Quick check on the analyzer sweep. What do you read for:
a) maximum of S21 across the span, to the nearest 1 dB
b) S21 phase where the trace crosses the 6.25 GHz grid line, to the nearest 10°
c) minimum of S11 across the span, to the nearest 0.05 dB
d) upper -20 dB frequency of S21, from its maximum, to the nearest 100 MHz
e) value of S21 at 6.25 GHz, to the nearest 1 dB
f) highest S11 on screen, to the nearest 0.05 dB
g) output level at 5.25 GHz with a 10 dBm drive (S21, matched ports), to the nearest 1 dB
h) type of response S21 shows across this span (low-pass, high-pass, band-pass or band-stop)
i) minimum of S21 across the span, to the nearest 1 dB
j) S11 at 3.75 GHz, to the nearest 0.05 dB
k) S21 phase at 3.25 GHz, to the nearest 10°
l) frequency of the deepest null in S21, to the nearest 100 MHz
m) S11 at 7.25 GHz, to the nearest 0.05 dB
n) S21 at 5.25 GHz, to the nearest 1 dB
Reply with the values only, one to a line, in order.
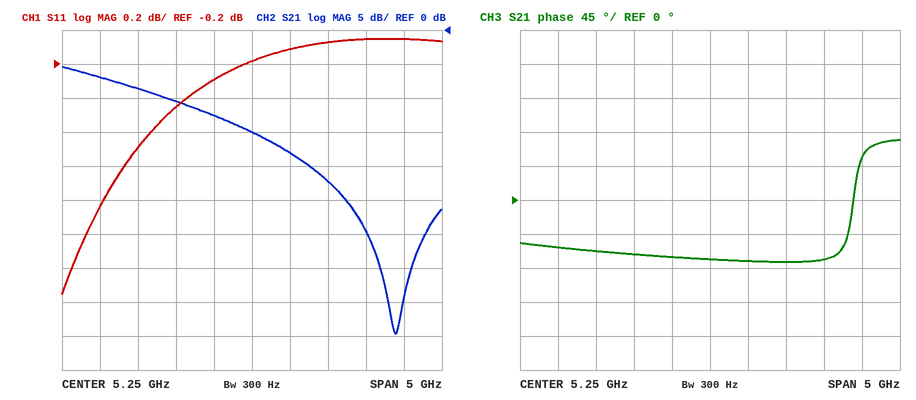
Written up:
-5 dB
-80°
-1.55 dB
6.5 GHz
-22 dB
-0.05 dB
-5 dBm
low-pass
-45 dB
-0.70 dB
-60°
7.1 GHz
-0.05 dB
-15 dB
